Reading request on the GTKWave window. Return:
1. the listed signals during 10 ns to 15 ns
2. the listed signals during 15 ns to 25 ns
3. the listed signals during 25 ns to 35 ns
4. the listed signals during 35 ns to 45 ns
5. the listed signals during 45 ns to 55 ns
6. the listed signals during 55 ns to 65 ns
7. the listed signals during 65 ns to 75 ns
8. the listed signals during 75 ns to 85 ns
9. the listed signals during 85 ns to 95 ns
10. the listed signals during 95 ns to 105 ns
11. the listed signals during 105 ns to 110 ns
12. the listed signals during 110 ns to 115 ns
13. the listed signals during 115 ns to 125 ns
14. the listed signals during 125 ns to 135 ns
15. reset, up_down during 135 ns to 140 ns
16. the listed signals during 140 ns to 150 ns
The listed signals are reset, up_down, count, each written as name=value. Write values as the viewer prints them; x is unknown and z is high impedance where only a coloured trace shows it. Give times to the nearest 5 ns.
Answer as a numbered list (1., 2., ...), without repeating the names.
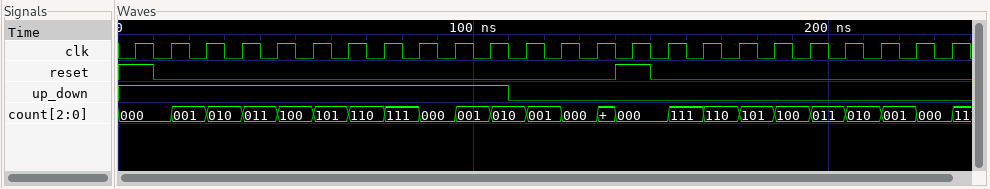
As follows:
1. reset=0, up_down=1, count=000
2. reset=0, up_down=1, count=001
3. reset=0, up_down=1, count=010
4. reset=0, up_down=1, count=011
5. reset=0, up_down=1, count=100
6. reset=0, up_down=1, count=101
7. reset=0, up_down=1, count=110
8. reset=0, up_down=1, count=111
9. reset=0, up_down=1, count=000
10. reset=0, up_down=1, count=001
11. reset=0, up_down=1, count=010
12. reset=0, up_down=0, count=010
13. reset=0, up_down=0, count=001
14. reset=0, up_down=0, count=000
15. reset=0, up_down=0
16. reset=1, up_down=0, count=000
